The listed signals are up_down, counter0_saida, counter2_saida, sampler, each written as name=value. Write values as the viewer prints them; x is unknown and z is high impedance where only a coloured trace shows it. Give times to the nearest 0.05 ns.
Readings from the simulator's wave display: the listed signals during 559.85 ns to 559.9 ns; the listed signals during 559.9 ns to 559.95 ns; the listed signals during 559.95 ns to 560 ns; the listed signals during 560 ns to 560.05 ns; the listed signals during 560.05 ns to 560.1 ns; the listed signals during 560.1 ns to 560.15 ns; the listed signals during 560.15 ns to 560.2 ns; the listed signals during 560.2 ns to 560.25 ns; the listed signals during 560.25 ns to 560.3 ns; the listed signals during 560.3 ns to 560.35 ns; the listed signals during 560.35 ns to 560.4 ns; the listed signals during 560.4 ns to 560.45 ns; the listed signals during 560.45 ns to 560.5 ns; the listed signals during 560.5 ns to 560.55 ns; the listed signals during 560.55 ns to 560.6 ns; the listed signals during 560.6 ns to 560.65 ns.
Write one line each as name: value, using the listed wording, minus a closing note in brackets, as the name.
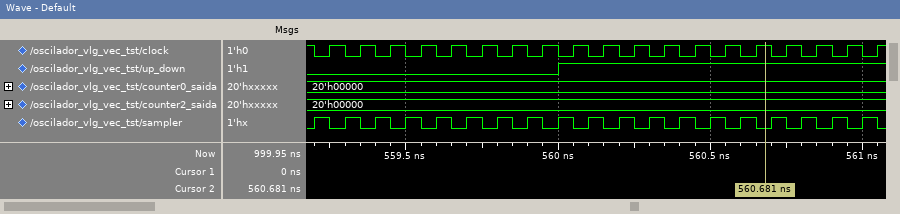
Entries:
the listed signals during 559.85 ns to 559.9 ns: up_down=0, counter0_saida=20'h00000, counter2_saida=20'h00000, sampler=0
the listed signals during 559.9 ns to 559.95 ns: up_down=0, counter0_saida=20'h00000, counter2_saida=20'h00000, sampler=1
the listed signals during 559.95 ns to 560 ns: up_down=0, counter0_saida=20'h00000, counter2_saida=20'h00000, sampler=0
the listed signals during 560 ns to 560.05 ns: up_down=1, counter0_saida=20'h00000, counter2_saida=20'h00000, sampler=1
the listed signals during 560.05 ns to 560.1 ns: up_down=1, counter0_saida=20'h00000, counter2_saida=20'h00000, sampler=0
the listed signals during 560.1 ns to 560.15 ns: up_down=1, counter0_saida=20'h00000, counter2_saida=20'h00000, sampler=1
the listed signals during 560.15 ns to 560.2 ns: up_down=1, counter0_saida=20'h00000, counter2_saida=20'h00000, sampler=0
the listed signals during 560.2 ns to 560.25 ns: up_down=1, counter0_saida=20'h00000, counter2_saida=20'h00000, sampler=1
the listed signals during 560.25 ns to 560.3 ns: up_down=1, counter0_saida=20'h00000, counter2_saida=20'h00000, sampler=0
the listed signals during 560.3 ns to 560.35 ns: up_down=1, counter0_saida=20'h00000, counter2_saida=20'h00000, sampler=1
the listed signals during 560.35 ns to 560.4 ns: up_down=1, counter0_saida=20'h00000, counter2_saida=20'h00000, sampler=0
the listed signals during 560.4 ns to 560.45 ns: up_down=1, counter0_saida=20'h00000, counter2_saida=20'h00000, sampler=1
the listed signals during 560.45 ns to 560.5 ns: up_down=1, counter0_saida=20'h00000, counter2_saida=20'h00000, sampler=0
the listed signals during 560.5 ns to 560.55 ns: up_down=1, counter0_saida=20'h00000, counter2_saida=20'h00000, sampler=1
the listed signals during 560.55 ns to 560.6 ns: up_down=1, counter0_saida=20'h00000, counter2_saida=20'h00000, sampler=0
the listed signals during 560.6 ns to 560.65 ns: up_down=1, counter0_saida=20'h00000, counter2_saida=20'h00000, sampler=1
